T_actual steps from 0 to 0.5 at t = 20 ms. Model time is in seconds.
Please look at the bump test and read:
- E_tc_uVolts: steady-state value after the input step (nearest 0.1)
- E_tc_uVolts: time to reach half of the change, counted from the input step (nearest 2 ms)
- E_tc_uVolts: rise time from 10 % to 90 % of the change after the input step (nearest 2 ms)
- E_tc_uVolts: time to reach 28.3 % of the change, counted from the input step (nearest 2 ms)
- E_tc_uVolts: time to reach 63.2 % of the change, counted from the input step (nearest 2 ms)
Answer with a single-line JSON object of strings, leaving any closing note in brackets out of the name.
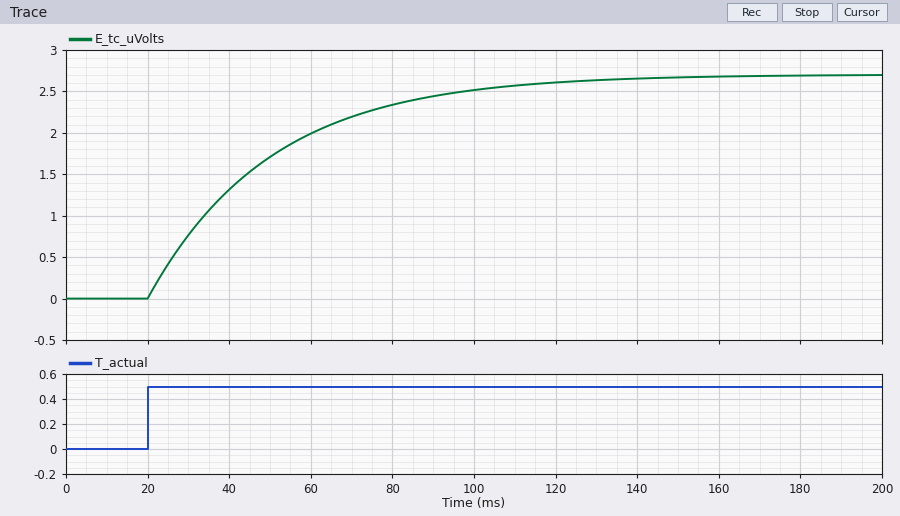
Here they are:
{"E_tc_uVolts: steady-state value after the input step": "2.7", "E_tc_uVolts: time to reach half of the change, counted from the input step": "20 ms", "E_tc_uVolts: rise time from 10 % to 90 % of the change after the input step": "66 ms", "E_tc_uVolts: time to reach 28.3 % of the change, counted from the input step": "10 ms", "E_tc_uVolts: time to reach 63.2 % of the change, counted from the input step": "30 ms"}
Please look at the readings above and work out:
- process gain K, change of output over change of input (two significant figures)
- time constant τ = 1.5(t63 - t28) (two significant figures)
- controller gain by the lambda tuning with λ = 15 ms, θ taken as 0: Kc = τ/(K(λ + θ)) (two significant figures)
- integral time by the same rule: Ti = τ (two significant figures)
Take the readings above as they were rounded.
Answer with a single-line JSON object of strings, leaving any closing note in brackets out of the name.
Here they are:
{"process gain K, change of output over change of input": "5.4", "time constant τ = 1.5(t63 - t28)": "30 ms", "controller gain by the lambda tuning with λ = 15 ms, θ taken as 0: Kc = τ/(K(λ + θ))": "0.37", "integral time by the same rule: Ti = τ": "30 ms"}
